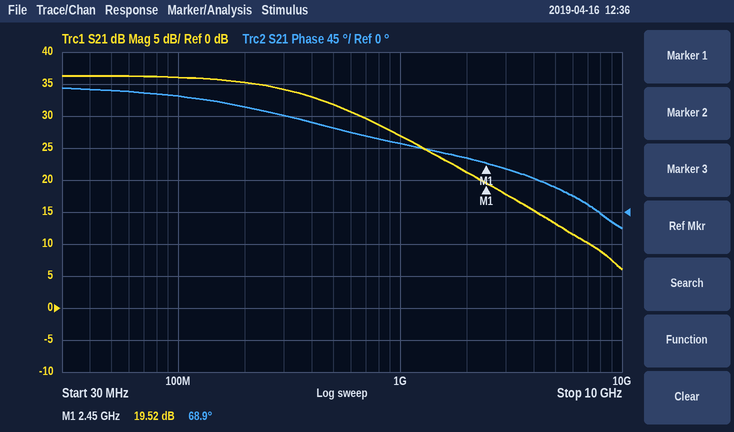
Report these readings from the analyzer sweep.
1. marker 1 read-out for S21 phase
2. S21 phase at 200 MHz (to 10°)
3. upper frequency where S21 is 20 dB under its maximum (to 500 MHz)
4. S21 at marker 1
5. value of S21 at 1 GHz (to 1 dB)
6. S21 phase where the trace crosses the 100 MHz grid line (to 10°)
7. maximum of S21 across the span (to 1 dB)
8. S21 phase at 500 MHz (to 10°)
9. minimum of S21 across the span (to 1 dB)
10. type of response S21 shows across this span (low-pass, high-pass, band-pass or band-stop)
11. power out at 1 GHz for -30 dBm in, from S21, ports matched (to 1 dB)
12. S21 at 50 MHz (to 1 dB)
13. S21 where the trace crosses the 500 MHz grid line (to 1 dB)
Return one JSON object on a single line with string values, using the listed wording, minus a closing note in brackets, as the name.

{"marker 1 read-out for S21 phase": "68.9°", "S21 phase at 200 MHz": "150°", "upper frequency where S21 is 20 dB under its maximum": "3.5 GHz", "S21 at marker 1": "19.52 dB", "value of S21 at 1 GHz": "27 dB", "S21 phase where the trace crosses the 100 MHz grid line": "160°", "maximum of S21 across the span": "36 dB", "S21 phase at 500 MHz": "120°", "minimum of S21 across the span": "6 dB", "type of response S21 shows across this span": "low-pass", "power out at 1 GHz for -30 dBm in, from S21, ports matched": "-3 dBm", "S21 at 50 MHz": "36 dB", "S21 where the trace crosses the 500 MHz grid line": "32 dB"}
